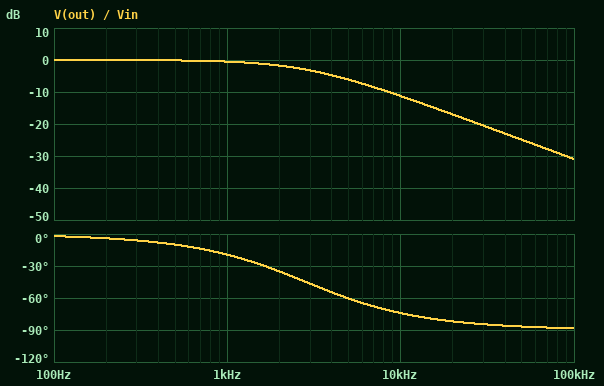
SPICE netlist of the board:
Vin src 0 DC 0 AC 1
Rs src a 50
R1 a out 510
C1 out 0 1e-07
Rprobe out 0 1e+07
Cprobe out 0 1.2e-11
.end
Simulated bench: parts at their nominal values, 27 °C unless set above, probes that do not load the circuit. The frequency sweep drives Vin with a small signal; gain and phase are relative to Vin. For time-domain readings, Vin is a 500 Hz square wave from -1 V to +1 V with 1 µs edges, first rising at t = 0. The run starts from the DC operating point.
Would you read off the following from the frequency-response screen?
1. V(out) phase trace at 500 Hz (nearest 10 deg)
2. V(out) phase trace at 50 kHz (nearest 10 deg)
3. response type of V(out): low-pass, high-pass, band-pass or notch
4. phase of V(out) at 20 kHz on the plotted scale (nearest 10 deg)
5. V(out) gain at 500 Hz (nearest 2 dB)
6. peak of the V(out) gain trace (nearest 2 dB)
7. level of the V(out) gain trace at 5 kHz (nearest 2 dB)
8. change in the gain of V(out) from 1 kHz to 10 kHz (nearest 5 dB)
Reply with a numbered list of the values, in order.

1. -10 deg
2. -90 deg
3. low-pass
4. -80 deg
5. 0 dB
6. 0 dB
7. -6 dB
8. -10 dB
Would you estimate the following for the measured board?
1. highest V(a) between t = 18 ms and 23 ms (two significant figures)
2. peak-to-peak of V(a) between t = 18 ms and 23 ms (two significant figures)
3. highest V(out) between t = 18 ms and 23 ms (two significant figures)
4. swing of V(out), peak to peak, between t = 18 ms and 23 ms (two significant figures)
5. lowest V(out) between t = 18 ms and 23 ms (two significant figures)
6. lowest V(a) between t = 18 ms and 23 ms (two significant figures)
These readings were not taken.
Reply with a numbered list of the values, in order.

1. 1.0 V
2. 2.0 V
3. 1.0 V
4. 2.0 V
5. -1.0 V
6. -1.0 V
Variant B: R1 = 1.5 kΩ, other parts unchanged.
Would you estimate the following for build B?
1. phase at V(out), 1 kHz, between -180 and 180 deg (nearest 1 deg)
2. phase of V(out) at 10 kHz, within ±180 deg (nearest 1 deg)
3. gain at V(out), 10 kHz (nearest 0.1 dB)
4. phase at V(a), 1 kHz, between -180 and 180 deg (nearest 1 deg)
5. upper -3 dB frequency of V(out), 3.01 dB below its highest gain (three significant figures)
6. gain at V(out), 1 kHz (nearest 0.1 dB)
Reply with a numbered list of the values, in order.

1. -44 deg
2. -84 deg
3. -19.8 dB
4. -1 deg
5. 1.03 kHz
6. -2.9 dB
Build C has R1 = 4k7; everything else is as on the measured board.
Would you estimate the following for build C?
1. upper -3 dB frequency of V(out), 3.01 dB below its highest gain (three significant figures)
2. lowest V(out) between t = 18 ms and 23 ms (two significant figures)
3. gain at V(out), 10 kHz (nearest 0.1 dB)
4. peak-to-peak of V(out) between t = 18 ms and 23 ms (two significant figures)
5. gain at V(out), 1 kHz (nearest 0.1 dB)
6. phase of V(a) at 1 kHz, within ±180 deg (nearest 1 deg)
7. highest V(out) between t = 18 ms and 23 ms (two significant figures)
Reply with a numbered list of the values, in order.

1. 335 Hz
2. -780 mV
3. -29.5 dB
4. 1.6 V
5. -10.0 dB
6. 0 deg
7. 780 mV
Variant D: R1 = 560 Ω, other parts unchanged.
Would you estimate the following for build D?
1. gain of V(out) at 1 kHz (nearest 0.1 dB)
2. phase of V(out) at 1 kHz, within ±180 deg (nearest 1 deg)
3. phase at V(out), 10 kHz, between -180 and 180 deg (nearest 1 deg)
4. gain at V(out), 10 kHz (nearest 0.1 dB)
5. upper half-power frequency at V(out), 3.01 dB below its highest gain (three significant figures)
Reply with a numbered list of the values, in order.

1. -0.6 dB
2. -21 deg
3. -75 deg
4. -12.0 dB
5. 2.61 kHz
